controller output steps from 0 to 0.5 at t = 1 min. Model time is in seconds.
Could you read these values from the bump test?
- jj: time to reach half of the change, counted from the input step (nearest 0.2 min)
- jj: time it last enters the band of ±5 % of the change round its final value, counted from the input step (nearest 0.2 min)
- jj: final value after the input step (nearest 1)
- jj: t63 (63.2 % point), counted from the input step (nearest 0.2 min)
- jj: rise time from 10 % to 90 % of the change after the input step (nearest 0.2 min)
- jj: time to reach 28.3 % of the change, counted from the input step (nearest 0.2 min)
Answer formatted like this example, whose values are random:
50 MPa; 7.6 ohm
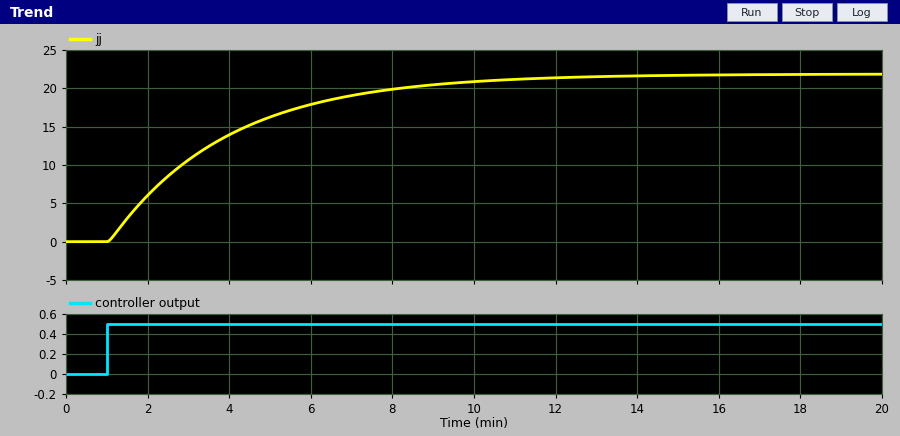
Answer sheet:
2.0 min; 8.8 min; 22; 3.0 min; 6.4 min; 1.0 min
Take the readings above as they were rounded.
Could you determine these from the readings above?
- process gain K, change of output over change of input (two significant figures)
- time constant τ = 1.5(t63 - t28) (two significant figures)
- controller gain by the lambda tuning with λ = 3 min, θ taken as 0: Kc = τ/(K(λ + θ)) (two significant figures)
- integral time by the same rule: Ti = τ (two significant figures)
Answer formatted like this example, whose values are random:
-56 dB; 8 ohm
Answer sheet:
44; 3.0 min; 0.023; 3.0 min
